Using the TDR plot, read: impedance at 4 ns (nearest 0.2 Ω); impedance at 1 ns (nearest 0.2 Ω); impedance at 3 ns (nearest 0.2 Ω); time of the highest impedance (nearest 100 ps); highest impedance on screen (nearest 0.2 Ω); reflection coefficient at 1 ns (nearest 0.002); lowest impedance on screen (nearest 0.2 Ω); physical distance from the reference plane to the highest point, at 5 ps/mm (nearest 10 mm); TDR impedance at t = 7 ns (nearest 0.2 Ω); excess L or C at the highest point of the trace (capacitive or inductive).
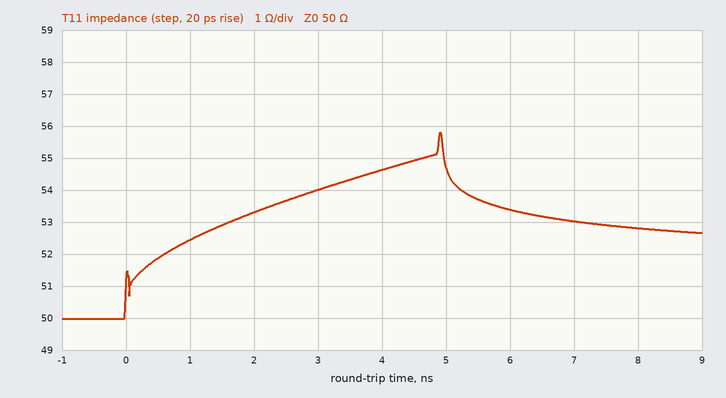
54.6 Ω
52.4 Ω
54.0 Ω
4.9 ns
55.8 Ω
+0.024
50.0 Ω
490 mm
53.0 Ω
inductive
